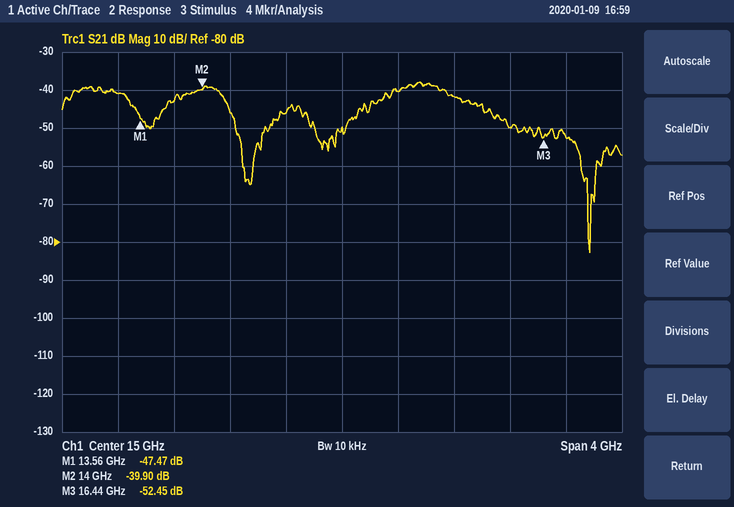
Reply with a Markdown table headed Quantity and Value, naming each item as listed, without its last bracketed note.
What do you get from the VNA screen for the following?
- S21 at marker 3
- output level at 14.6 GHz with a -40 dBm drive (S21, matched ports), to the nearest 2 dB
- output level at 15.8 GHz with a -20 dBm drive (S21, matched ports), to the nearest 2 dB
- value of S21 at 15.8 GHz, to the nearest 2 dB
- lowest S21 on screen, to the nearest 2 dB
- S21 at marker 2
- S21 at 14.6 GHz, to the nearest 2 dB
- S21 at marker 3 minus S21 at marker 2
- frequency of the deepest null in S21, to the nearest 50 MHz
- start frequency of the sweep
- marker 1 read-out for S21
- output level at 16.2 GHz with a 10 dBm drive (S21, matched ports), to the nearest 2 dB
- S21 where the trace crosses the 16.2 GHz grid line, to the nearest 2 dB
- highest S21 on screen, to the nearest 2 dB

| Quantity | Value |
|---|---|
| S21 at marker 3 | -52.45 dB |
| output level at 14.6 GHz with a -40 dBm drive (S21, matched ports), to the nearest 2 dB | -86 dBm |
| output level at 15.8 GHz with a -20 dBm drive (S21, matched ports), to the nearest 2 dB | -62 dBm |
| value of S21 at 15.8 GHz, to the nearest 2 dB | -42 dB |
| lowest S21 on screen, to the nearest 2 dB | -82 dB |
| S21 at marker 2 | -39.90 dB |
| S21 at 14.6 GHz, to the nearest 2 dB | -46 dB |
| S21 at marker 3 minus S21 at marker 2 | -12.55 dB |
| frequency of the deepest null in S21, to the nearest 50 MHz | 16.75 GHz |
| start frequency of the sweep | 13 GHz |
| marker 1 read-out for S21 | -47.47 dB |
| output level at 16.2 GHz with a 10 dBm drive (S21, matched ports), to the nearest 2 dB | -40 dBm |
| S21 where the trace crosses the 16.2 GHz grid line, to the nearest 2 dB | -50 dB |
| highest S21 on screen, to the nearest 2 dB | -38 dB |
